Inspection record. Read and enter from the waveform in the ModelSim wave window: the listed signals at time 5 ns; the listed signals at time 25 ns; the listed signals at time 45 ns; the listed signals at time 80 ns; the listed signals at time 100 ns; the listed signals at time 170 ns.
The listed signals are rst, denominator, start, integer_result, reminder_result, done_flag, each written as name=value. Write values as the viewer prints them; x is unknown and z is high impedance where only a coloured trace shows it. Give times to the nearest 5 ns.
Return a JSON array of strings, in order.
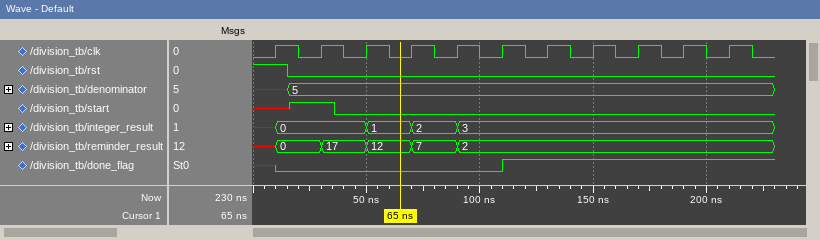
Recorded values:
["rst=1, denominator=x, start=x, integer_result=x, reminder_result=x, done_flag=x", "rst=0, denominator=5, start=1, integer_result=0, reminder_result=0, done_flag=0", "rst=0, denominator=5, start=0, integer_result=0, reminder_result=17, done_flag=0", "rst=0, denominator=5, start=0, integer_result=2, reminder_result=7, done_flag=0", "rst=0, denominator=5, start=0, integer_result=3, reminder_result=2, done_flag=0", "rst=0, denominator=5, start=0, integer_result=3, reminder_result=2, done_flag=1"]
